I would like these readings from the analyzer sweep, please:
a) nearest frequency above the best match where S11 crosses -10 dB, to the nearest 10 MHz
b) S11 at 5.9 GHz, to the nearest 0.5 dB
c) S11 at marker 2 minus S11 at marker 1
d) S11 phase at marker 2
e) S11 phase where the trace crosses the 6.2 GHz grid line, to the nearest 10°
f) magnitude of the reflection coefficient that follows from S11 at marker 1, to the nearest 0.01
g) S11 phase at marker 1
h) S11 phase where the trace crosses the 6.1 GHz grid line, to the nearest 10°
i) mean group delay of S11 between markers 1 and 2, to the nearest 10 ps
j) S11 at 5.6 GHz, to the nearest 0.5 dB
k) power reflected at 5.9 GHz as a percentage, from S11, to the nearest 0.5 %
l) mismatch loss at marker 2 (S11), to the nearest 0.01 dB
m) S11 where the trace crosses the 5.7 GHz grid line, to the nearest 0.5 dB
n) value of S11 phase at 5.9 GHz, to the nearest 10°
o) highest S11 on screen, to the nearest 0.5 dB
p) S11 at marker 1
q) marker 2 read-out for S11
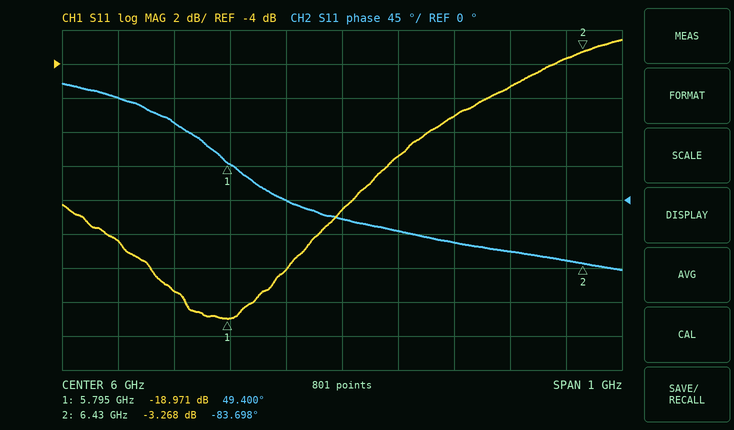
6.08 GHz
-16.0 dB
15.703 dB
-83.698°
-60°
0.11
49.400°
-40°
580 ps
-14.5 dB
2.5 %
2.77 dB
-17.5 dB
0°
-2.5 dB
-18.971 dB
-3.268 dB
